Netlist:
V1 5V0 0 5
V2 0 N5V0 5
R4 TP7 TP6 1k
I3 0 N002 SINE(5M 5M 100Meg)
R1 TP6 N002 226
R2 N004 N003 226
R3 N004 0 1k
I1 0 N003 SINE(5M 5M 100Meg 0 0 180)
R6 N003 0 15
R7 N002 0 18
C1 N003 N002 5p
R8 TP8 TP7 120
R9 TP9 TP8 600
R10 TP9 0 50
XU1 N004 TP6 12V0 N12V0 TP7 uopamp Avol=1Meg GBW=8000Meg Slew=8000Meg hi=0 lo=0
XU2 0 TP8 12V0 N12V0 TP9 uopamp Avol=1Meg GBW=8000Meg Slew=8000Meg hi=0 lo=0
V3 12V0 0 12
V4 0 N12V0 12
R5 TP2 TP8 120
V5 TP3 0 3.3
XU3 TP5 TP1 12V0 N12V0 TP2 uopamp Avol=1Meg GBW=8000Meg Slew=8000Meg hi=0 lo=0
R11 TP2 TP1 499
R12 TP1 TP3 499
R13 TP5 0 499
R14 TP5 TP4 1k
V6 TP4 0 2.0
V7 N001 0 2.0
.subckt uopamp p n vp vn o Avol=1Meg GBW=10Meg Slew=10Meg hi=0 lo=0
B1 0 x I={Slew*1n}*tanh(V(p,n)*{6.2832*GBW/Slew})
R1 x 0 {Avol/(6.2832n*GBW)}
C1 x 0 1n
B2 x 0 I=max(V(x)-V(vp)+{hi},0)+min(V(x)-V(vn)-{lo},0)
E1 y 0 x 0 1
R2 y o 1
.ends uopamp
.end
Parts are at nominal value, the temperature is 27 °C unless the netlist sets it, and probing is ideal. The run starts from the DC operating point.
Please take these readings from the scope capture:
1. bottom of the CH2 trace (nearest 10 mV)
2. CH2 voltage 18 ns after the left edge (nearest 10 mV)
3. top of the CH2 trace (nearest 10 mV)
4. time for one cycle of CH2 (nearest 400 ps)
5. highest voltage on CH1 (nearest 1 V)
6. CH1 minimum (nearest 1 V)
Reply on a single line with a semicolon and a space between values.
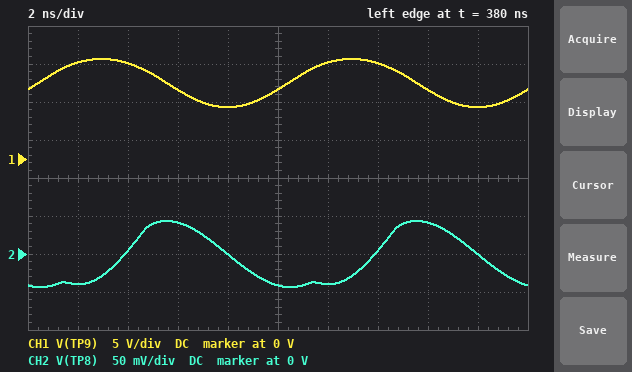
-40 mV; 0 V; 40 mV; 10.0 ns; 13 V; 7 V
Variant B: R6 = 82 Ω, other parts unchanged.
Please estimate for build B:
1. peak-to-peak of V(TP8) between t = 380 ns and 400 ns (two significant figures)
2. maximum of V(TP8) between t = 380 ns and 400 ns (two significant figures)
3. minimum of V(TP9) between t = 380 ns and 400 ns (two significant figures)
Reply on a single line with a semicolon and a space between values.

300 mV; 150 mV; -5.7 V
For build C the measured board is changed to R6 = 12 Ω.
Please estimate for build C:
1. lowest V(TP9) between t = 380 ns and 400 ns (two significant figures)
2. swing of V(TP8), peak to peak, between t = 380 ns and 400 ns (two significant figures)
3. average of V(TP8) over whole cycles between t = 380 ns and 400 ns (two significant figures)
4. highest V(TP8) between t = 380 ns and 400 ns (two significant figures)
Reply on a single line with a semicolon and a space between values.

7.4 V; 79 mV; -6.9 mV; 39 mV
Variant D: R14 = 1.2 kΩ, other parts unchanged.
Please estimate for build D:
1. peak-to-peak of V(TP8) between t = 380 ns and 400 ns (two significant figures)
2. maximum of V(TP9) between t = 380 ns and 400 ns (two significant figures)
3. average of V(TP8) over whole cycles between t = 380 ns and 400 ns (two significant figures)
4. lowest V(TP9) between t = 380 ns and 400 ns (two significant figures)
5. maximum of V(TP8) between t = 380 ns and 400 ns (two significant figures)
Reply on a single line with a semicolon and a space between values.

96 mV; 14 V; -12 mV; 7.6 V; 43 mV
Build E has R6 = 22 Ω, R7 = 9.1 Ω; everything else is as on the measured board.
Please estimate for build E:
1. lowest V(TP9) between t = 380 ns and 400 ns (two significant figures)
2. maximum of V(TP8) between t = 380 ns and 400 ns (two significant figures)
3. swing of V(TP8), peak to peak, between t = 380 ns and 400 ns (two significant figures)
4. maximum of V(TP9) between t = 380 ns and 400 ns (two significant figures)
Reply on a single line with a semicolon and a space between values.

5.3 V; 42 mV; 84 mV; 12 V
